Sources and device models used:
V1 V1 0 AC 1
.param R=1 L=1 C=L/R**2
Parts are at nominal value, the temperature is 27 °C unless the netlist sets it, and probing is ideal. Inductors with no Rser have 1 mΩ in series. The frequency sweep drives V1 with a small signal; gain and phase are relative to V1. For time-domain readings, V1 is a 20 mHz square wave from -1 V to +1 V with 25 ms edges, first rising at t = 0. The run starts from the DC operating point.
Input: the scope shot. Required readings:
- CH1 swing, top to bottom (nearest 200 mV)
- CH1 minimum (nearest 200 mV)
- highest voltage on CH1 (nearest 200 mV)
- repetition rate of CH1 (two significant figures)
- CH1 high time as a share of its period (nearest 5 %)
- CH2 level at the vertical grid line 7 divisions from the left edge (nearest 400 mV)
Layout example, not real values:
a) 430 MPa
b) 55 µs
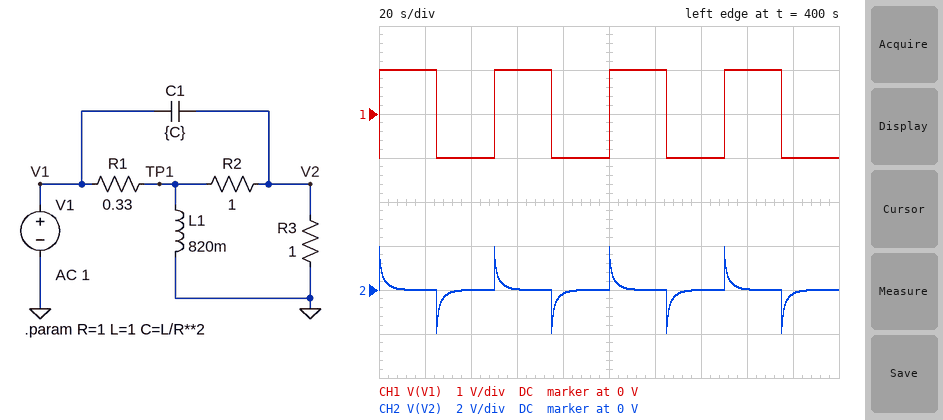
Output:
a) 2.0 V
b) -1.0 V
c) 1.0 V
d) 20 mHz
e) 50 %
f) 0 V
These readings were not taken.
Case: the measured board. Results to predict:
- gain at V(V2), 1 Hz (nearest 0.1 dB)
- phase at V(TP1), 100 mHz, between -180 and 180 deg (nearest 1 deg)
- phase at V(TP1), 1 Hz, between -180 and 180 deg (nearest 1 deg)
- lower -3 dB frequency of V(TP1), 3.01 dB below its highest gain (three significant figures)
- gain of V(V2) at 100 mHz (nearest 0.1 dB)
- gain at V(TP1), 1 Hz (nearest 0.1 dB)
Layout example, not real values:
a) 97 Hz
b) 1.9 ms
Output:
a) -0.2 dB
b) 32 deg
c) 5 deg
d) 73.6 mHz
e) -4.6 dB
f) -0.1 dB
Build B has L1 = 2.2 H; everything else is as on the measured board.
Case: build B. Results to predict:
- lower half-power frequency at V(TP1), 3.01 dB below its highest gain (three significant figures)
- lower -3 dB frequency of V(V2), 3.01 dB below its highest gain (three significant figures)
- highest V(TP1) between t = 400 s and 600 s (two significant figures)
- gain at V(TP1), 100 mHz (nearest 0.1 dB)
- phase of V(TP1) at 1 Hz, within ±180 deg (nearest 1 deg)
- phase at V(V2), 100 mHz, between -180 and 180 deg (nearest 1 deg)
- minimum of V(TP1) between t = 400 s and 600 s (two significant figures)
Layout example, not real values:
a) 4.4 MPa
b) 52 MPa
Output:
a) 29.1 mHz
b) 199 mHz
c) 1.9 V
d) -1.3 dB
e) 3 deg
f) 28 deg
g) -1.9 V
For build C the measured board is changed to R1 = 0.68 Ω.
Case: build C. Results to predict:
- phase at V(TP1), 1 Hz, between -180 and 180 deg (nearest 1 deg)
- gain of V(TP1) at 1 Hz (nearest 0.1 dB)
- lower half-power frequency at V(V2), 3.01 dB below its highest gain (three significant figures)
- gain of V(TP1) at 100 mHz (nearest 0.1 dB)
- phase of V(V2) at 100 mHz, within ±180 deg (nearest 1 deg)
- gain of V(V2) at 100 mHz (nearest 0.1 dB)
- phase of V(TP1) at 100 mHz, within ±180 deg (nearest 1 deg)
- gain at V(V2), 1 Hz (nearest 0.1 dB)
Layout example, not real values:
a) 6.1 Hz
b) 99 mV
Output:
a) 8 deg
b) -0.1 dB
c) 159 mHz
d) -4.6 dB
e) 54 deg
f) -5.2 dB
g) 52 deg
h) -0.1 dB
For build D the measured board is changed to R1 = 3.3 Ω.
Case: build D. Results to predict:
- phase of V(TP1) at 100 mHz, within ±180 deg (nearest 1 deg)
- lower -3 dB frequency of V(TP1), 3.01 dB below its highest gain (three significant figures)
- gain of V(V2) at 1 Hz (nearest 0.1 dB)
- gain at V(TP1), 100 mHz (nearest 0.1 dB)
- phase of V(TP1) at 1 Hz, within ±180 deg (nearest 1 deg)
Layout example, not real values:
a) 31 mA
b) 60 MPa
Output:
a) 101 deg
b) 234 mHz
c) 0 dB
d) -12.2 dB
e) 16 deg
